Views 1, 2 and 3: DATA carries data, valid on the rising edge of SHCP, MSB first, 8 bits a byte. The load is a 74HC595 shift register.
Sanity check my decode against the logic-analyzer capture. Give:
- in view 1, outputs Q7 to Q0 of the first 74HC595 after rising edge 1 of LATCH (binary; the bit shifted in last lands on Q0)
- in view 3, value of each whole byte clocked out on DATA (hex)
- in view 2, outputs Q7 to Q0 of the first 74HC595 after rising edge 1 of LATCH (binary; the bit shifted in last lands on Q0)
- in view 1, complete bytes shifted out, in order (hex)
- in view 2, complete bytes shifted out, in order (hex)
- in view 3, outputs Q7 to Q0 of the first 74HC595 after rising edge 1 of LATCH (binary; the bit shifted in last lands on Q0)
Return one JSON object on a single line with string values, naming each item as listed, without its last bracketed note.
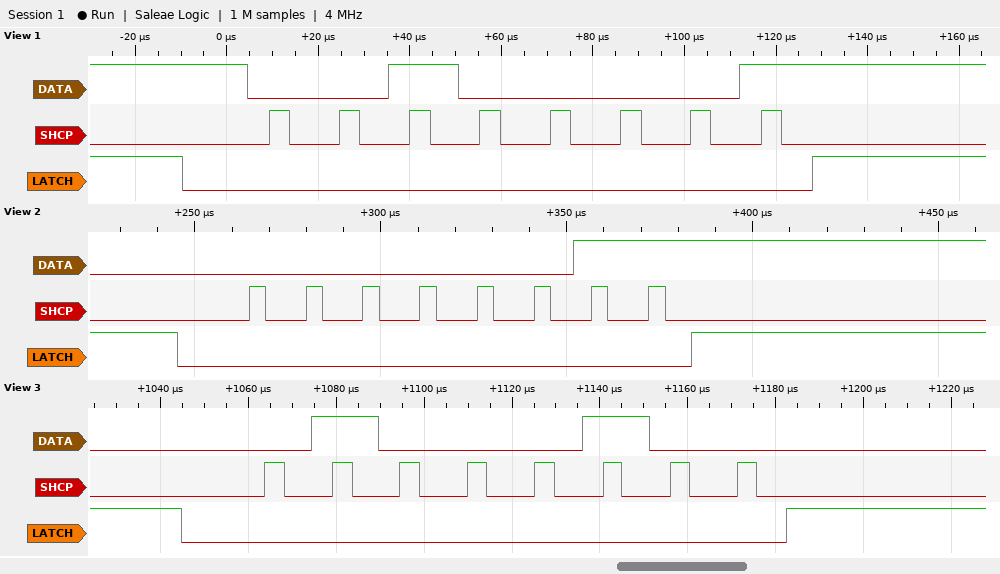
{"in view 1, outputs Q7 to Q0 of the first 74HC595 after rising edge 1 of LATCH": "00100001", "in view 3, value of each whole byte clocked out on DATA": "44", "in view 2, outputs Q7 to Q0 of the first 74HC595 after rising edge 1 of LATCH": "00000011", "in view 1, complete bytes shifted out, in order": "21", "in view 2, complete bytes shifted out, in order": "03", "in view 3, outputs Q7 to Q0 of the first 74HC595 after rising edge 1 of LATCH": "01000100"}
